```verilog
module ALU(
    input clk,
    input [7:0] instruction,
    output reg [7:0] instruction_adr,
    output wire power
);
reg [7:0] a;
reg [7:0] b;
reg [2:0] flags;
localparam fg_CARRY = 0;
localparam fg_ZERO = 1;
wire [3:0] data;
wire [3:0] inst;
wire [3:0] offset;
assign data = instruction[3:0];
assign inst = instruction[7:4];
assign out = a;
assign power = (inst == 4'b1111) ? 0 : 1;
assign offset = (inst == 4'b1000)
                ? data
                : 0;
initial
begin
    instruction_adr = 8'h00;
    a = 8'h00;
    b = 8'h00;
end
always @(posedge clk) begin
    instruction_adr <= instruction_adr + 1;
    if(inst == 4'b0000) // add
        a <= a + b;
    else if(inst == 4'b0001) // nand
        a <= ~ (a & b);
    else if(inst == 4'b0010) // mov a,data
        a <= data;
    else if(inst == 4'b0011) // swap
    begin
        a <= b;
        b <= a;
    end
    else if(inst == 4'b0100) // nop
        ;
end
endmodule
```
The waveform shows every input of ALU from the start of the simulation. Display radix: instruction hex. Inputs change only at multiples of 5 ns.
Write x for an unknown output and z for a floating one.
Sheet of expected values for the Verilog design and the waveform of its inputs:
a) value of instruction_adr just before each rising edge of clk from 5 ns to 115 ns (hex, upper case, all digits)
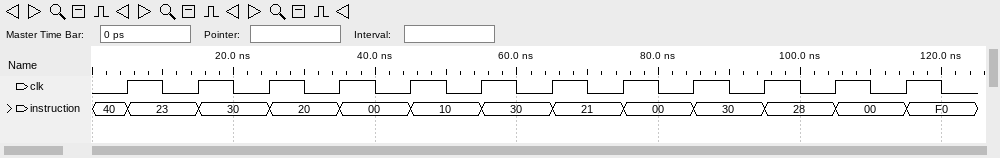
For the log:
00, 01, 02, 03, 04, 05, 06, 07, 08, 09, 0A, 0B
